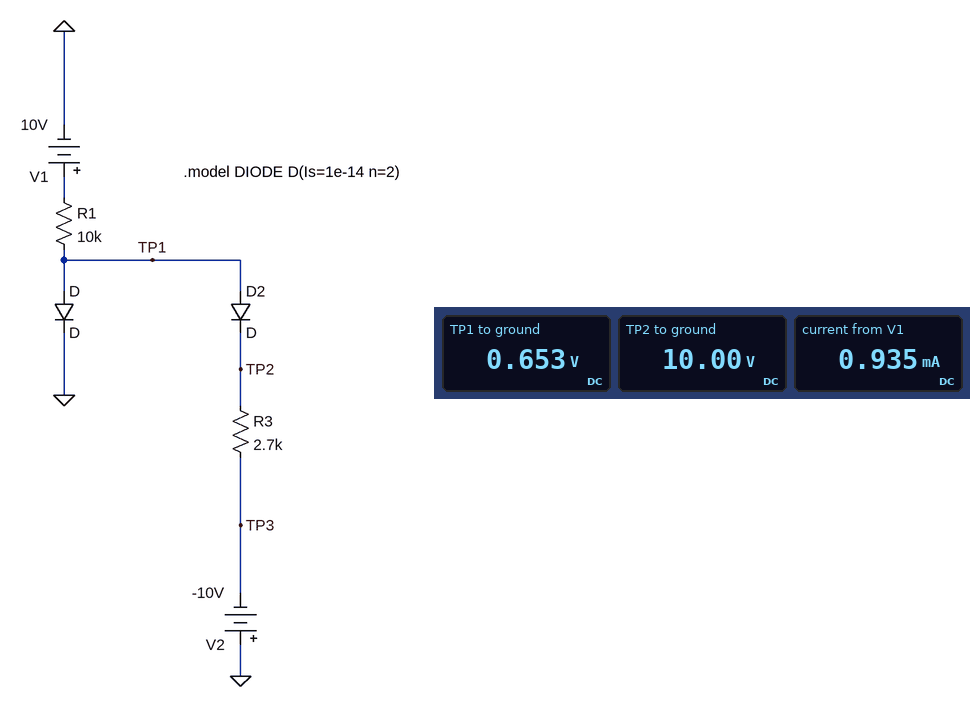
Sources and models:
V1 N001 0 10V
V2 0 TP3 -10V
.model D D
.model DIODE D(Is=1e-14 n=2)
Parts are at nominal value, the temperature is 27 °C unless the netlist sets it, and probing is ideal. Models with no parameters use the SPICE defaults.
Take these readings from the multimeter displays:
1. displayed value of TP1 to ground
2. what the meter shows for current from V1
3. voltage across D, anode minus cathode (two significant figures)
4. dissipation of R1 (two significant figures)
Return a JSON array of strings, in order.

["0.653 V", "0.935 mA", "650 mV", "8.7 mW"]
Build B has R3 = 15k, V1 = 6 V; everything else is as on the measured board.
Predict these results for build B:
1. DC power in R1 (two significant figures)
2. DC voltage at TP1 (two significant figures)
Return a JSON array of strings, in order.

["2.9 mW", "640 mV"]
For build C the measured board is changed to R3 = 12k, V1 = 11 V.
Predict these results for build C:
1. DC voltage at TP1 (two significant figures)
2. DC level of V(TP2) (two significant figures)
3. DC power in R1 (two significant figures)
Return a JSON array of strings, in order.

["660 mV", "10 V", "11 mW"]
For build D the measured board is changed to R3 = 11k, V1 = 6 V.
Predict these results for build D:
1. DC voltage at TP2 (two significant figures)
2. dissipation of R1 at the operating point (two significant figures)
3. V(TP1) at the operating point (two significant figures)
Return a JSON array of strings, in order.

["10 V", "2.9 mW", "640 mV"]
